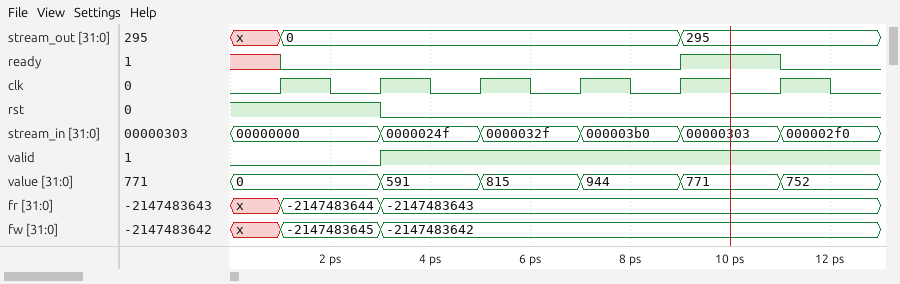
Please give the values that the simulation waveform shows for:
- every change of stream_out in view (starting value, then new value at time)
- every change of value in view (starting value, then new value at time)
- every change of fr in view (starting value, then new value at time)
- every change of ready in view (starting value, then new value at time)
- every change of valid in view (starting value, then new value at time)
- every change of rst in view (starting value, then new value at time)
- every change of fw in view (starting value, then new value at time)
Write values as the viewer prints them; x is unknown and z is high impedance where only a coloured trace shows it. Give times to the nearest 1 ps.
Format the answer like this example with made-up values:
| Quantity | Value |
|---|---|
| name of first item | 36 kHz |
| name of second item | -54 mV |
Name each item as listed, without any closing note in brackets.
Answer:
| Quantity | Value |
|---|---|
| every change of stream_out in view | x, 0 at 1 ps, 295 at 9 ps |
| every change of value in view | 0, 591 at 3 ps, 815 at 5 ps, 944 at 7 ps, 771 at 9 ps, 752 at 11 ps |
| every change of fr in view | x, -2147483644 at 1 ps, -2147483643 at 3 ps |
| every change of ready in view | x, 0 at 1 ps, 1 at 9 ps, 0 at 11 ps |
| every change of valid in view | 0, 1 at 3 ps |
| every change of rst in view | 1, 0 at 3 ps |
| every change of fw in view | x, -2147483645 at 1 ps, -2147483642 at 3 ps |
